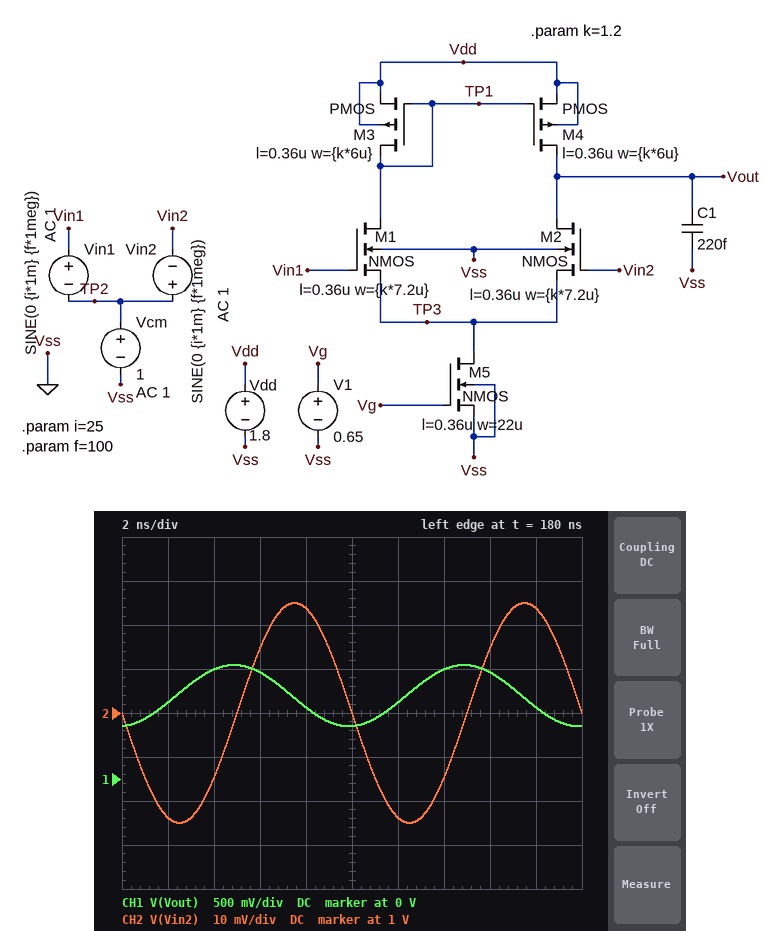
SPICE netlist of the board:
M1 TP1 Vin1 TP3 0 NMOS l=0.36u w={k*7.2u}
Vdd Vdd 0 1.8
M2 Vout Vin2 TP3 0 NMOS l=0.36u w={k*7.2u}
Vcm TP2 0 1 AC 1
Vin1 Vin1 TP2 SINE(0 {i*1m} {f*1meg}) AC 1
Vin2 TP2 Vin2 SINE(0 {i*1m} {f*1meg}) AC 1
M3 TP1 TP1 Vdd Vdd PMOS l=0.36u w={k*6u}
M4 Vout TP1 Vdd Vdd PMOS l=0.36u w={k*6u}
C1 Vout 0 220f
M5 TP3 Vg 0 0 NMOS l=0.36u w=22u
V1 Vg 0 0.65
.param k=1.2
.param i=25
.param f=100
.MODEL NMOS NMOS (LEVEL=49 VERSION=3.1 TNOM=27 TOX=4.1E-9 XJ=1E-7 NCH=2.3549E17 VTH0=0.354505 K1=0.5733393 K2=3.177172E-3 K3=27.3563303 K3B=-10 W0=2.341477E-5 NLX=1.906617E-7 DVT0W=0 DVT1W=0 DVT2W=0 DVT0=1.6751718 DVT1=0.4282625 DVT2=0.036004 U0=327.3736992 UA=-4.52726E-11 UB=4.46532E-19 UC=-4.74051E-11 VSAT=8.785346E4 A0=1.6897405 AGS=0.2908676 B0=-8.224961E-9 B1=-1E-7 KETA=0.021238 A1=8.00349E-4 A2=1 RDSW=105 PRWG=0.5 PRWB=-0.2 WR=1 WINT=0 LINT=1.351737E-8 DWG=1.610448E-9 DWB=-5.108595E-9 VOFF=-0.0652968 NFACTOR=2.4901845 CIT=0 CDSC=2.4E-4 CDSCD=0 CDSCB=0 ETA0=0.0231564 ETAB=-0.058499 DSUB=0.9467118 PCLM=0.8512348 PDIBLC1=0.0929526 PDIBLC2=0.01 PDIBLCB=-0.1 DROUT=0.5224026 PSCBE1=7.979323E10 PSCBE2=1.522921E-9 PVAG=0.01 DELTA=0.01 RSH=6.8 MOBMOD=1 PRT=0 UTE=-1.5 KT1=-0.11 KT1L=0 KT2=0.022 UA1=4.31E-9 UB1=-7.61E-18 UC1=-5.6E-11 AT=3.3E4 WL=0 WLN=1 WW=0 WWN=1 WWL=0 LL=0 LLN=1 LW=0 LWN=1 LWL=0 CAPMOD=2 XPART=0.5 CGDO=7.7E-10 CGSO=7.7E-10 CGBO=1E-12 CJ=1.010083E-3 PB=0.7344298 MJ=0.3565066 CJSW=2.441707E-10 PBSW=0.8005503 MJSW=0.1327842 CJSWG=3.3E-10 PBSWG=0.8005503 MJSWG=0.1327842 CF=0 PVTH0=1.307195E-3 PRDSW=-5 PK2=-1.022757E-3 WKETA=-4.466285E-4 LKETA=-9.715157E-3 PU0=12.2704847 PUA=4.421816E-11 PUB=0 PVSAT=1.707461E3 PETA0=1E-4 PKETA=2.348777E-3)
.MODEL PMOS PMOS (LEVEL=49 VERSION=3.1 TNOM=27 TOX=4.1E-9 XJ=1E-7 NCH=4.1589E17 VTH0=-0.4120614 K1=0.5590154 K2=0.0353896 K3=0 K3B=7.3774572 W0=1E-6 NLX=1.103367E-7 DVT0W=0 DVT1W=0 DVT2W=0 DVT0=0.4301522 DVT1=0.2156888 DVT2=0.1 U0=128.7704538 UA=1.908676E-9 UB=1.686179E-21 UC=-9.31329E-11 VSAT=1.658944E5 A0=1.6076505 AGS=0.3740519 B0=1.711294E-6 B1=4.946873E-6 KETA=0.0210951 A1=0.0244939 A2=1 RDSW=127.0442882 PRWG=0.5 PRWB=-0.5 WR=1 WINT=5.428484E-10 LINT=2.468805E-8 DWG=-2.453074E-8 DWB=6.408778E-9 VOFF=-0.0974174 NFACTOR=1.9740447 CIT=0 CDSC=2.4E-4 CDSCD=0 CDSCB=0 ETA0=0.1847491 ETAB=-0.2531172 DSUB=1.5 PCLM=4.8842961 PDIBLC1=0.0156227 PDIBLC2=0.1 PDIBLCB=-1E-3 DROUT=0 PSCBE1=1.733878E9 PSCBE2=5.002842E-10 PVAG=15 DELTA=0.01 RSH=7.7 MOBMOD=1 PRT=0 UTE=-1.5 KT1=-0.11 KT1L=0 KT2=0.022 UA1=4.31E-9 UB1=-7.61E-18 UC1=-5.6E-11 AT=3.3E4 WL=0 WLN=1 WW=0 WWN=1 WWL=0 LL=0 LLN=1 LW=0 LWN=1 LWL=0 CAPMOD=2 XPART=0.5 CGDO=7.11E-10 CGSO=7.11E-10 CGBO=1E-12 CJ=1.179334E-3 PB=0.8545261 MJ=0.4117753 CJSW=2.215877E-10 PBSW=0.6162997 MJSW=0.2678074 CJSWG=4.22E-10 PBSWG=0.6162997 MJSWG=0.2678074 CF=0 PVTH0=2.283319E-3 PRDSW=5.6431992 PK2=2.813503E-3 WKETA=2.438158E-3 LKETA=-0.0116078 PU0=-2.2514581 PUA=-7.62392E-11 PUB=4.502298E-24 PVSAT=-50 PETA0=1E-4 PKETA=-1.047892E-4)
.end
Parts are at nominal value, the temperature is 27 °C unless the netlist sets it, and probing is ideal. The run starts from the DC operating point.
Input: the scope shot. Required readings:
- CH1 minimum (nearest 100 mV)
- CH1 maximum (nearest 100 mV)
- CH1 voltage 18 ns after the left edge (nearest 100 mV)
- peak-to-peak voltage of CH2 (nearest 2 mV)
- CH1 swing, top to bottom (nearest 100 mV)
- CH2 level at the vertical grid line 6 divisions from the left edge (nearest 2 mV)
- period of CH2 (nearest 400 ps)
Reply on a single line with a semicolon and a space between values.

600 mV; 1.3 V; 800 mV; 50 mV; 700 mV; 976 mV; 10.0 ns
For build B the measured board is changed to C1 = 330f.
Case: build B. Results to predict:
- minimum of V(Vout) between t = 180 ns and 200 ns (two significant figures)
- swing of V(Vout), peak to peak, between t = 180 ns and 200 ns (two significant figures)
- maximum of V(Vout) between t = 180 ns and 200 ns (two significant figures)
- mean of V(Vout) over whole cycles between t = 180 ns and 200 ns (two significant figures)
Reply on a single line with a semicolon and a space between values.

700 mV; 480 mV; 1.2 V; 940 mV
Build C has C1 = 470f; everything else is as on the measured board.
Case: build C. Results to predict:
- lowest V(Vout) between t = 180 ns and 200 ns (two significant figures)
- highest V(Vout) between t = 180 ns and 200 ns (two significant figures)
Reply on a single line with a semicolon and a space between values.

770 mV; 1.1 V
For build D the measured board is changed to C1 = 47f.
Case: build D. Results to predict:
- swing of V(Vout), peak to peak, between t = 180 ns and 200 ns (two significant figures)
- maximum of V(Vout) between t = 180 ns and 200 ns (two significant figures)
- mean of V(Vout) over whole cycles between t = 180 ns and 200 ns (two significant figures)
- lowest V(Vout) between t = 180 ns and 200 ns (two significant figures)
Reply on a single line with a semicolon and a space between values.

1.3 V; 1.6 V; 990 mV; 340 mV
